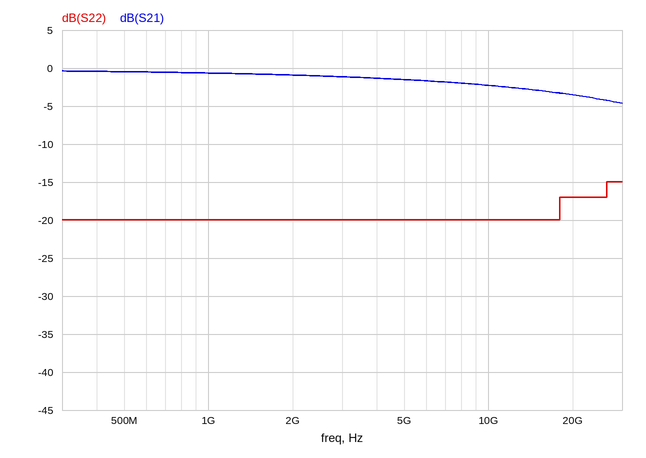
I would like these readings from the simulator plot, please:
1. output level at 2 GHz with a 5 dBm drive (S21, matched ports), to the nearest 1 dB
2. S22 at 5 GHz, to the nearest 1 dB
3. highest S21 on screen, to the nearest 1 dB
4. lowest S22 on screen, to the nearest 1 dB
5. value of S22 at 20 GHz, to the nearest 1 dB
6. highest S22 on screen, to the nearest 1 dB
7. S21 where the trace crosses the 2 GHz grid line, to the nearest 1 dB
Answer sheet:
4 dBm
-20 dB
0 dB
-20 dB
-17 dB
-15 dB
-1 dB
